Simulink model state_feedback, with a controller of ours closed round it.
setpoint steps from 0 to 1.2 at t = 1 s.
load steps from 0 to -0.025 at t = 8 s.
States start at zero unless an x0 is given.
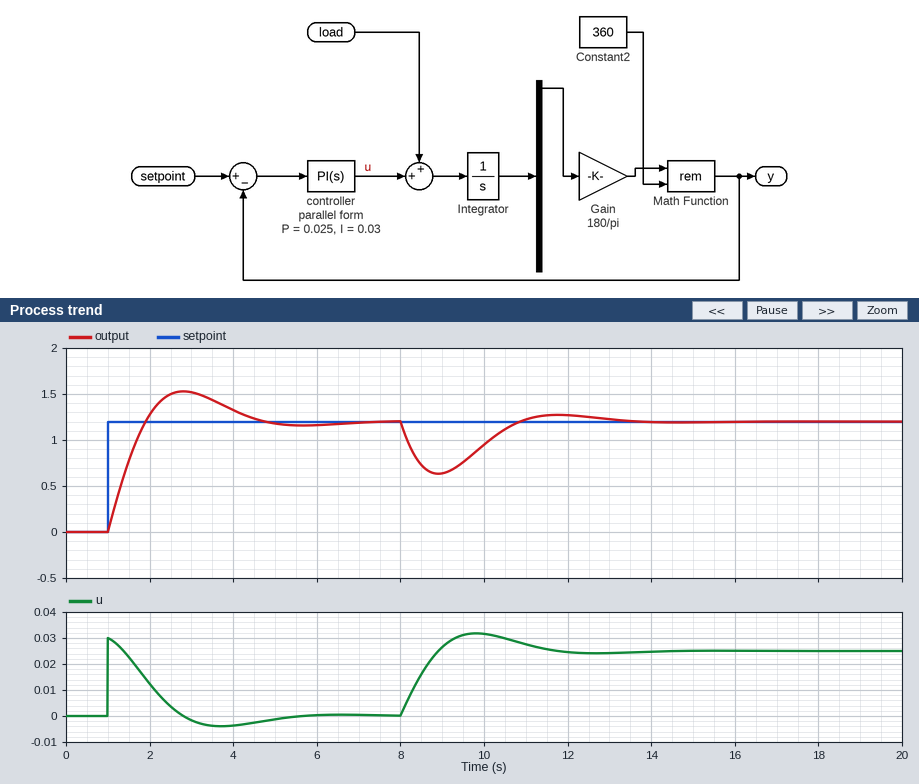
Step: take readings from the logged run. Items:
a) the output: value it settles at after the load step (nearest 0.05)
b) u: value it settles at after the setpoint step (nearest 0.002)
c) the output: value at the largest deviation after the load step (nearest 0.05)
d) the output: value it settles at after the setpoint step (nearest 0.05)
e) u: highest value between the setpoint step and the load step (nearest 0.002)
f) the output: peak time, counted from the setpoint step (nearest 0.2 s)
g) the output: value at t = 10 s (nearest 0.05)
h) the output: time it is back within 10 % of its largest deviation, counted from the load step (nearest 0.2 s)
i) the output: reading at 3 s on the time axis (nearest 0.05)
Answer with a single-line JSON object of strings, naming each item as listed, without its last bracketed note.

{"the output: value it settles at after the load step": "1.20", "u: value it settles at after the setpoint step": "0.000", "the output: value at the largest deviation after the load step": "0.65", "the output: value it settles at after the setpoint step": "1.20", "u: highest value between the setpoint step and the load step": "0.030", "the output: peak time, counted from the setpoint step": "1.8 s", "the output: value at t = 10 s": "0.95", "the output: time it is back within 10 % of its largest deviation, counted from the load step": "4.4 s", "the output: reading at 3 s on the time axis": "1.50"}
